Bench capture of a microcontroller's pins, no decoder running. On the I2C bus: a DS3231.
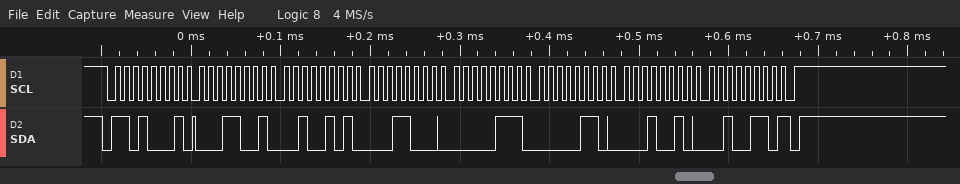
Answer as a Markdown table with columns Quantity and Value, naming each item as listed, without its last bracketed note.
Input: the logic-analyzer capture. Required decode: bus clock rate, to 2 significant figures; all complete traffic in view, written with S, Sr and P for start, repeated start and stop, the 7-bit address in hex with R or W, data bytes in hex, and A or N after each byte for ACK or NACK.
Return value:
| Quantity | Value |
|---|---|
| bus clock rate, to 2 significant figures | 100 kHz |
| all complete traffic in view, written with S, Sr and P for start, repeated start and stop, the 7-bit address in hex with R or W, data bytes in hex, and A or N after each byte for ACK or NACK | S 68R A 19 A 25 A 18 A 07 A 06 A 12 A 26 N P |
